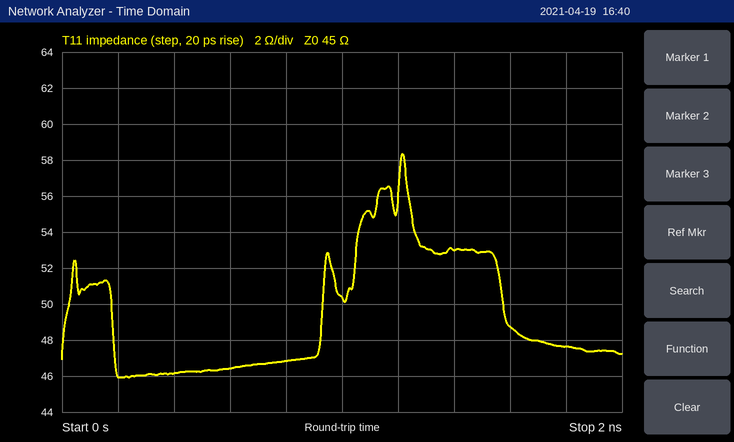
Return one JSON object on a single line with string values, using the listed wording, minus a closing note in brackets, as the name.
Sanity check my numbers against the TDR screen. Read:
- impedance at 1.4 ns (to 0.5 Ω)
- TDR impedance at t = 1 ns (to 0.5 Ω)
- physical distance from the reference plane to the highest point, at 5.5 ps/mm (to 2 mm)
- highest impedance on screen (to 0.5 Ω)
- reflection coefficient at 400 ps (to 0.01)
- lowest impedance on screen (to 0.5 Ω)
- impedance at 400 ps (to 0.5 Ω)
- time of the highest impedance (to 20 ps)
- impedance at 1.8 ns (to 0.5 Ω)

{"impedance at 1.4 ns": "53.0 Ω", "TDR impedance at t = 1 ns": "50.5 Ω", "physical distance from the reference plane to the highest point, at 5.5 ps/mm": "110 mm", "highest impedance on screen": "58.5 Ω", "reflection coefficient at 400 ps": "+0.01", "lowest impedance on screen": "46.0 Ω", "impedance at 400 ps": "46.0 Ω", "time of the highest impedance": "1.22 ns", "impedance at 1.8 ns": "47.5 Ω"}
